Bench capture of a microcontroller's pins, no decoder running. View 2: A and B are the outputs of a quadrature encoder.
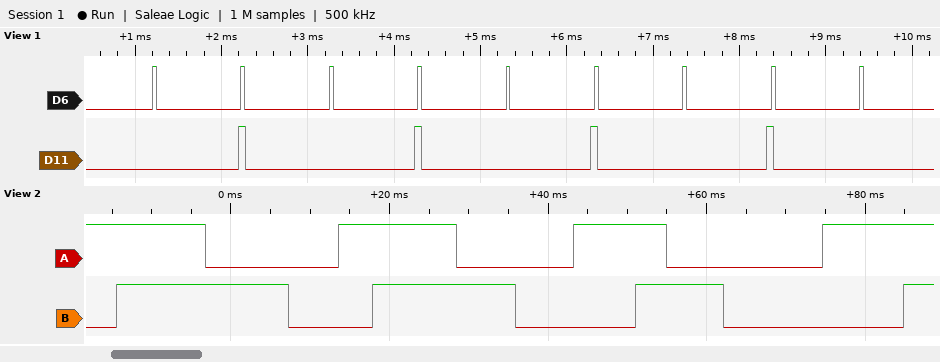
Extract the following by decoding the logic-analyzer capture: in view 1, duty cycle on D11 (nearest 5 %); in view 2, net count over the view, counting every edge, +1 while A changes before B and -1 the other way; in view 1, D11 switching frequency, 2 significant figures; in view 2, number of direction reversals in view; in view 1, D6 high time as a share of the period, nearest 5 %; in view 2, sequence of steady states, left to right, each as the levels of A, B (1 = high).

5 %
+13
490 Hz
0
5 %
10 11 01 00 10 11 01 00 10 11 01 00 10 11
